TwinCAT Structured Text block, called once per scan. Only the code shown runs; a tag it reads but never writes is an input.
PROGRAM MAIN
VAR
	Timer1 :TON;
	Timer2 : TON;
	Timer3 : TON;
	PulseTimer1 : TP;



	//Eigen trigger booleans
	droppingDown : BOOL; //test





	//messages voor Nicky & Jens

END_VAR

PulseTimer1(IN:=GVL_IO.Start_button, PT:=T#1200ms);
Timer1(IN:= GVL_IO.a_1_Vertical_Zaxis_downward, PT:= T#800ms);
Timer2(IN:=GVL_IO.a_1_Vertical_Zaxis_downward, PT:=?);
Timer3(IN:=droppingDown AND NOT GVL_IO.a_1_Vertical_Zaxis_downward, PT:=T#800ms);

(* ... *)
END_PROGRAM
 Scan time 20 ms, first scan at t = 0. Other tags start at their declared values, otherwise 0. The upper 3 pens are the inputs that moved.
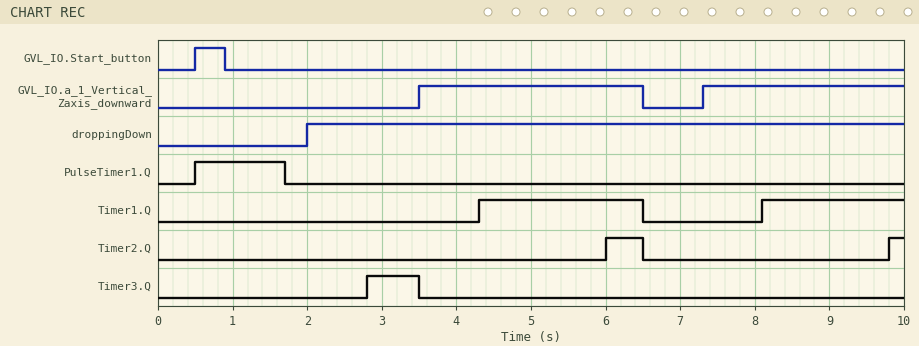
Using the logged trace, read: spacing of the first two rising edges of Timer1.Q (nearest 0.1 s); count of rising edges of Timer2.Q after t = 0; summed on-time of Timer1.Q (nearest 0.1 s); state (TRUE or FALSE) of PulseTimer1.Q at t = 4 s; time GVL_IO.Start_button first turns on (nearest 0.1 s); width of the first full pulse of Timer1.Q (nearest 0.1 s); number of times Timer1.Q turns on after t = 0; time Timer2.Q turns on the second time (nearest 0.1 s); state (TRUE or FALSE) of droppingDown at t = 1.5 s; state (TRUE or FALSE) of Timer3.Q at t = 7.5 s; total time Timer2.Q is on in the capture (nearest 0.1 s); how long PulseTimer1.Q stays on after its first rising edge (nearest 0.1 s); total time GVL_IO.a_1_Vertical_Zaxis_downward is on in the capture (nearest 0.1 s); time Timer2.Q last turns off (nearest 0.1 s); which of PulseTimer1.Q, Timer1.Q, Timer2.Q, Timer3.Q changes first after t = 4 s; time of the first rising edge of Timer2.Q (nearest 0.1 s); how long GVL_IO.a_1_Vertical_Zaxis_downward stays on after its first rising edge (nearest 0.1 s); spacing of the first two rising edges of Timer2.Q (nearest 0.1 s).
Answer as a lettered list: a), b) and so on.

a) 3.8 s
b) 2
c) 4.1 s
d) FALSE
e) 0.5 s
f) 2.2 s
g) 2
h) 9.8 s
i) FALSE
j) FALSE
k) 0.7 s
l) 1.2 s
m) 5.7 s
n) 6.5 s
o) Timer1.Q
p) 6.0 s
q) 3.0 s
r) 3.8 s
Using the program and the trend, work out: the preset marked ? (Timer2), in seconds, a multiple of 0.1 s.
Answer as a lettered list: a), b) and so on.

a) 2.5 s
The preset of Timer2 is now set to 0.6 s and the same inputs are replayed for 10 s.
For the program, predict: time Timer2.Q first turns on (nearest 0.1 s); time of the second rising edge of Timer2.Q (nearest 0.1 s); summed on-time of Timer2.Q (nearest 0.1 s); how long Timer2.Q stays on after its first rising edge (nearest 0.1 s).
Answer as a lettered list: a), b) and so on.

a) 4.1 s
b) 7.9 s
c) 4.5 s
d) 2.4 s
